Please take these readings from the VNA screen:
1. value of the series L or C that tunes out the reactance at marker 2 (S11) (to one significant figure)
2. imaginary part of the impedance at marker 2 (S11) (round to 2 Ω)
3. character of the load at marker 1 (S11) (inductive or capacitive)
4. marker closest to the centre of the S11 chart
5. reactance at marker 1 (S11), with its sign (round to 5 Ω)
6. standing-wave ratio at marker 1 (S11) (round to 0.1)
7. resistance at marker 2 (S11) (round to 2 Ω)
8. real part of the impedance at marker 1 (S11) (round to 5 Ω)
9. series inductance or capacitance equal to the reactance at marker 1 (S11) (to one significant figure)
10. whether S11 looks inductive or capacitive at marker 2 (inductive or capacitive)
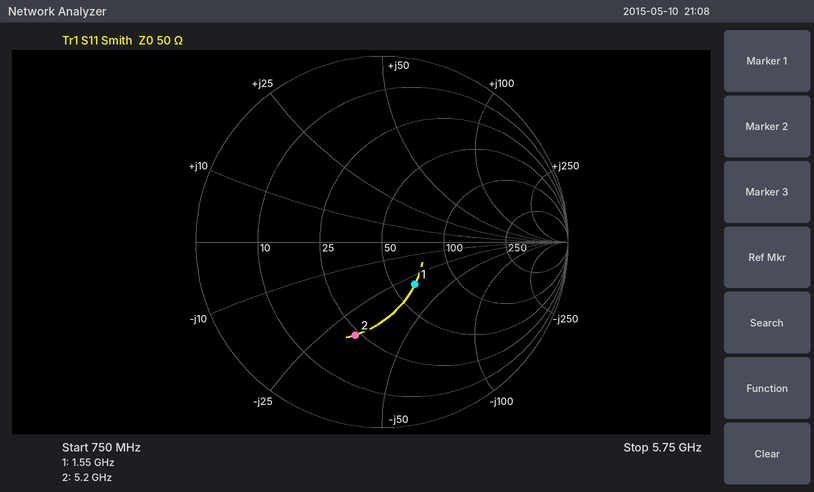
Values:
1.0 nH
-32 Ω
capacitive
marker 1
-30 Ω
1.8
24 Ω
65 Ω
3 pF
capacitive
